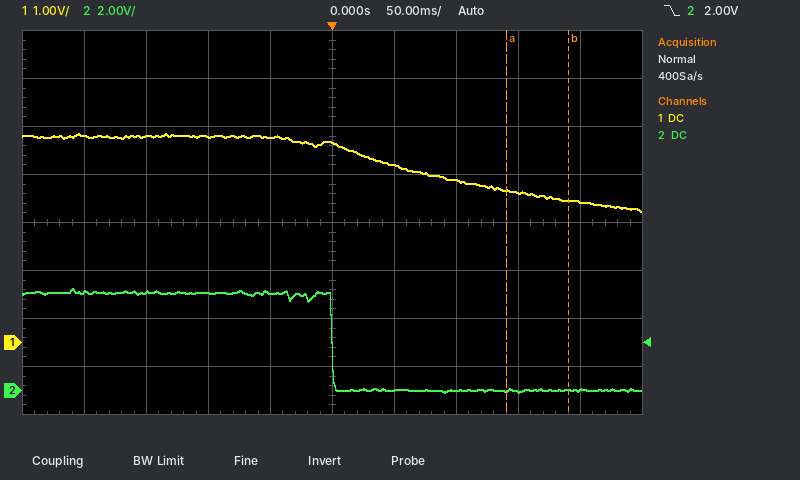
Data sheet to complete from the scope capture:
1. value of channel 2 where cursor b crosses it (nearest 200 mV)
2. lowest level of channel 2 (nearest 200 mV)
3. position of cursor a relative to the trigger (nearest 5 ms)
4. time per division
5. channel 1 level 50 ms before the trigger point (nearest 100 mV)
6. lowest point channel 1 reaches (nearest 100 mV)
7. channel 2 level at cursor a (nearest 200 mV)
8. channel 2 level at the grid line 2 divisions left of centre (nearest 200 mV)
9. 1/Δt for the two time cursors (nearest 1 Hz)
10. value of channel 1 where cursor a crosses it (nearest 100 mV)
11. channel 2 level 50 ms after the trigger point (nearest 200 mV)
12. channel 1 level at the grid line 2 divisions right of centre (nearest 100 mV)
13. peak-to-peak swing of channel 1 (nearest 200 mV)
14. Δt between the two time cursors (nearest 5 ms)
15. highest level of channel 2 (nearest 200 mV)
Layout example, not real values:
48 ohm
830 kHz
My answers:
0.0 V
0.0 V
+140 ms
50 ms
4.3 V
2.7 V
0.0 V
4.0 V
20 Hz
3.2 V
0.0 V
3.4 V
1.6 V
50 ms
4.2 V
